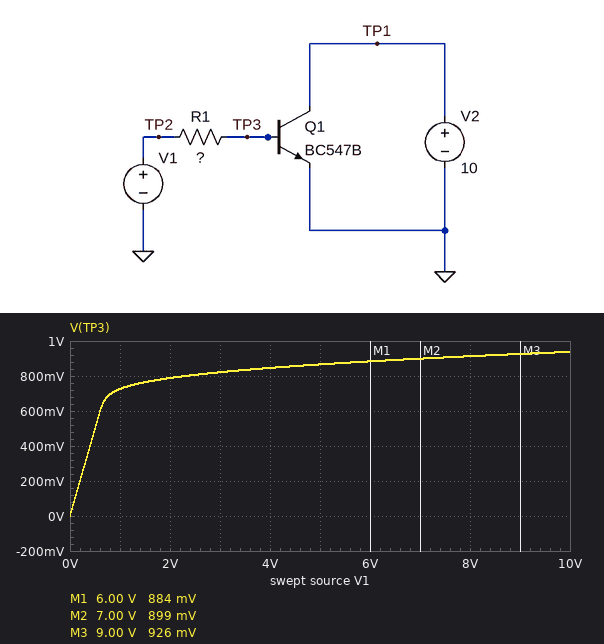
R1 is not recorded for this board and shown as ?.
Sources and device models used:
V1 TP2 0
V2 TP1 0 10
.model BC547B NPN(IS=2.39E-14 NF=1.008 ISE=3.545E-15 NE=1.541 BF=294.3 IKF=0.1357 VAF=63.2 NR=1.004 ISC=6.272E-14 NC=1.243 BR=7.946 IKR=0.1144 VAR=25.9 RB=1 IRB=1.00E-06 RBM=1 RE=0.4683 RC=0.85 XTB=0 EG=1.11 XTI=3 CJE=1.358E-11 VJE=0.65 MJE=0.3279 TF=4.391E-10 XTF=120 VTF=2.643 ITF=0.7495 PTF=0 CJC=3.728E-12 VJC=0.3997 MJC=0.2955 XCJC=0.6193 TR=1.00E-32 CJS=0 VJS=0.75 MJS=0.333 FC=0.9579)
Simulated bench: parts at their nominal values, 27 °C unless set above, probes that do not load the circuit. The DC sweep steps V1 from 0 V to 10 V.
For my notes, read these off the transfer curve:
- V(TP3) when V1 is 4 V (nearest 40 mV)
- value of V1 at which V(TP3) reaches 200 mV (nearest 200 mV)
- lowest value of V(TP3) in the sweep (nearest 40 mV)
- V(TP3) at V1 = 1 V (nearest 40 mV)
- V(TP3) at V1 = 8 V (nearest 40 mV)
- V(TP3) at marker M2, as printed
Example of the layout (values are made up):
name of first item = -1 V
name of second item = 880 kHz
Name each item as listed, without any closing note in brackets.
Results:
V(TP3) when V1 is 4 V = 840 mV
value of V1 at which V(TP3) reaches 200 mV = 200 mV
lowest value of V(TP3) in the sweep = 0 V
V(TP3) at V1 = 1 V = 720 mV
V(TP3) at V1 = 8 V = 920 mV
V(TP3) at marker M2, as printed = 899 mV
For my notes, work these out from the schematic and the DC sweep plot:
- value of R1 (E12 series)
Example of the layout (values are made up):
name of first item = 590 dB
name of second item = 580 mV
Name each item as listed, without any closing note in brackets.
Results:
value of R1 = 3.9 kΩ
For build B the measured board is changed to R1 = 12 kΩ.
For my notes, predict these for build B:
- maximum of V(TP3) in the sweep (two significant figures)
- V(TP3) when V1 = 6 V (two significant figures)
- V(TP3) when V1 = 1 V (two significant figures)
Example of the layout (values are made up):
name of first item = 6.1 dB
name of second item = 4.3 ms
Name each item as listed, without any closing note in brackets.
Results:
maximum of V(TP3) in the sweep = 840 mV
V(TP3) when V1 = 6 V = 810 mV
V(TP3) when V1 = 1 V = 690 mV
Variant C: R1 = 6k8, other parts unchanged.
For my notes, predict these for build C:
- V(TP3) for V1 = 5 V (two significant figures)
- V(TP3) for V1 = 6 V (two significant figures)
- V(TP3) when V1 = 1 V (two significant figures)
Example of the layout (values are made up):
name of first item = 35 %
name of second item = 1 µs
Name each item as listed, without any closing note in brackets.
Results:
V(TP3) for V1 = 5 V = 830 mV
V(TP3) for V1 = 6 V = 840 mV
V(TP3) when V1 = 1 V = 710 mV
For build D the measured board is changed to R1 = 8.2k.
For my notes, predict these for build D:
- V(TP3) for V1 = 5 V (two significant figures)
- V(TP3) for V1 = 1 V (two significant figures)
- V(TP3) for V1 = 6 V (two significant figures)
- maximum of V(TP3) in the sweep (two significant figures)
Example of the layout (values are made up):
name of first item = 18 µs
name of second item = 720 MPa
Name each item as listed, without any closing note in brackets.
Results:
V(TP3) for V1 = 5 V = 820 mV
V(TP3) for V1 = 1 V = 700 mV
V(TP3) for V1 = 6 V = 830 mV
maximum of V(TP3) in the sweep = 870 mV
